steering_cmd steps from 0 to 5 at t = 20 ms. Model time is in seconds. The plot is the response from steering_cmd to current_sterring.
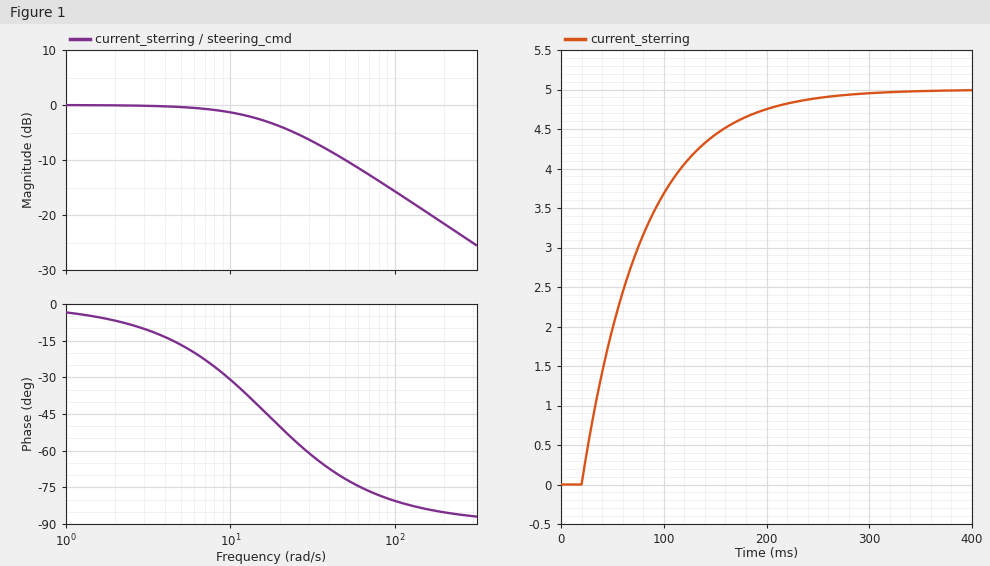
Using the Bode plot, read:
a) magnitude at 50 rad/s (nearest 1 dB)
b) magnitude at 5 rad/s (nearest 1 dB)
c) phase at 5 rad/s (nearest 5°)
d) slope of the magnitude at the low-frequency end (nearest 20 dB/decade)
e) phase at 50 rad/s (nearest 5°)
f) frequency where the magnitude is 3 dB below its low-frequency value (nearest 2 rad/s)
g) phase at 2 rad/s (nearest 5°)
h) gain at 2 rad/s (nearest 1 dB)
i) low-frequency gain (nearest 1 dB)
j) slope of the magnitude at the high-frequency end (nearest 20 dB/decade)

-10 dB
0 dB
-15°
0 dB/decade
-70°
16 rad/s
-5°
0 dB
0 dB
-20 dB/decade
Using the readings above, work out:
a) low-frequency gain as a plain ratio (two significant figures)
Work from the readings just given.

1.0
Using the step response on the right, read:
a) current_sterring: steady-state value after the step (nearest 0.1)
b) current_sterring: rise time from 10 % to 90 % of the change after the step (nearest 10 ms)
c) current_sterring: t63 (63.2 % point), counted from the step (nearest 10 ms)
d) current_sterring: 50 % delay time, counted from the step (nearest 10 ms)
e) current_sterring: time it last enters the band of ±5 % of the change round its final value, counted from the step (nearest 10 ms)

5.0
130 ms
60 ms
40 ms
180 ms
